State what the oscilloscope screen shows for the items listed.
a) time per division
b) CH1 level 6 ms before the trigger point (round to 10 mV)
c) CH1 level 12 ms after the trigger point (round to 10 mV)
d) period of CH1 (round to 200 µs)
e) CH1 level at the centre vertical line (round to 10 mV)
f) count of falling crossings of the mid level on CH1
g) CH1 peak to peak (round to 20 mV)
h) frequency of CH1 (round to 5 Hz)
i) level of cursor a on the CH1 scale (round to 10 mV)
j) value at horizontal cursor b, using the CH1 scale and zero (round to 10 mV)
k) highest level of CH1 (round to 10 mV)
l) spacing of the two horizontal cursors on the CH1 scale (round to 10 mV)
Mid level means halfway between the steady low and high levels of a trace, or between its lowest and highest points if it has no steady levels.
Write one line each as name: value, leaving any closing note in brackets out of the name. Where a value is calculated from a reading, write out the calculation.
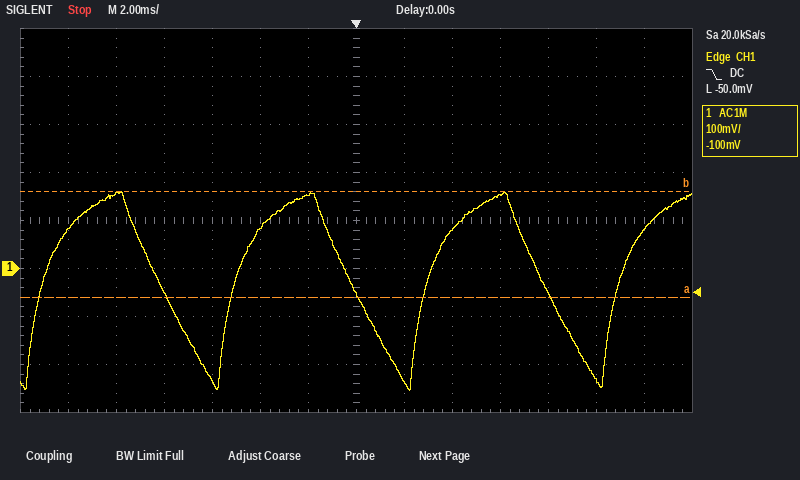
time per division: 2 ms
CH1 level 6 ms before the trigger point: -230 mV
CH1 level 12 ms after the trigger point: 80 mV
period of CH1: 8.0 ms
CH1 level at the centre vertical line: -50 mV
count of falling crossings of the mid level on CH1: 3
CH1 peak to peak: 420 mV
frequency of CH1: 1 / 8.0 ms ≈ 125 Hz
level of cursor a on the CH1 scale: -60 mV
value at horizontal cursor b, using the CH1 scale and zero: 160 mV
highest level of CH1: 160 mV
spacing of the two horizontal cursors on the CH1 scale: 220 mV
